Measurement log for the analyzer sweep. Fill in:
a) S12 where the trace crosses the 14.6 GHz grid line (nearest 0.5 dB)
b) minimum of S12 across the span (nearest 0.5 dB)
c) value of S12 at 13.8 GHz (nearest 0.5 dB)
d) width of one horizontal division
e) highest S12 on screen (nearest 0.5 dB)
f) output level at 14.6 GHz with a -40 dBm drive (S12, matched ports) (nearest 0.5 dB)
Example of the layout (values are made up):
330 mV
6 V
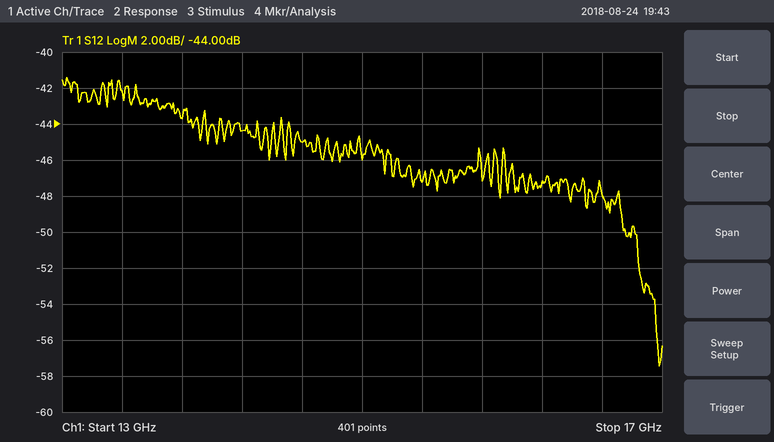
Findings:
-45.0 dB
-57.5 dB
-43.5 dB
400 MHz
-41.5 dB
-85.0 dBm
